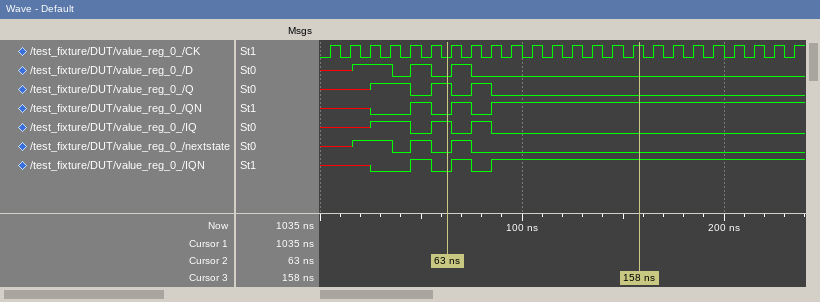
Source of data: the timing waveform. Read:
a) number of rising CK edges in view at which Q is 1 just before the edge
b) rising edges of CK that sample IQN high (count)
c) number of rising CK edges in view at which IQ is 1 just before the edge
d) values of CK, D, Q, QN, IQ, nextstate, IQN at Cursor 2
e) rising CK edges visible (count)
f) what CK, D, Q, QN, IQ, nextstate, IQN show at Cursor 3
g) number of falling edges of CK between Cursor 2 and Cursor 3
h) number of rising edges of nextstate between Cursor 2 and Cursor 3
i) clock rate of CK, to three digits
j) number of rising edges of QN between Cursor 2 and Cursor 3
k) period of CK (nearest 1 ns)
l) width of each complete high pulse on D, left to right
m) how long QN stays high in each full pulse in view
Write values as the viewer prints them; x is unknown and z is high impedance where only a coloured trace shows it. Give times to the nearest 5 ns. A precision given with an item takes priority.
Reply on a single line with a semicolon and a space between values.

4; 17; 4; CK=0, D=0, Q=1, QN=0, IQ=1, nextstate=0, IQN=0; 24; CK=1, D=0, Q=0, QN=1, IQ=0, nextstate=0, IQN=1; 9; 1; 100 MHz; 2; 10 ns; 10 ns, 10 ns; 10 ns, 10 ns
